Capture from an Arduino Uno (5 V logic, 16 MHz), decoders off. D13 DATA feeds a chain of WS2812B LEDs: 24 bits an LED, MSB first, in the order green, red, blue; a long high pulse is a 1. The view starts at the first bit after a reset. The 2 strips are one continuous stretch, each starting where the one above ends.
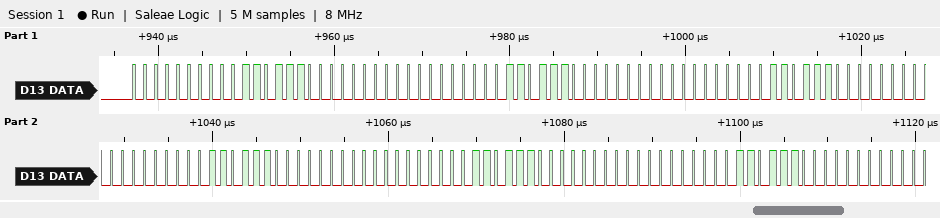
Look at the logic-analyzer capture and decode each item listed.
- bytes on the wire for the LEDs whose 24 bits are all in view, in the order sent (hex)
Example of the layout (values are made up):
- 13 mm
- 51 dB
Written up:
- 00 37 00 00 37 00 00 37 00 00 37 00 00 37 00 00 37 00
